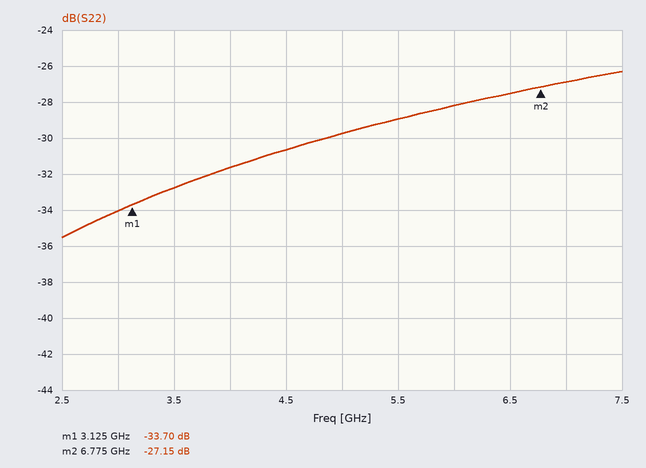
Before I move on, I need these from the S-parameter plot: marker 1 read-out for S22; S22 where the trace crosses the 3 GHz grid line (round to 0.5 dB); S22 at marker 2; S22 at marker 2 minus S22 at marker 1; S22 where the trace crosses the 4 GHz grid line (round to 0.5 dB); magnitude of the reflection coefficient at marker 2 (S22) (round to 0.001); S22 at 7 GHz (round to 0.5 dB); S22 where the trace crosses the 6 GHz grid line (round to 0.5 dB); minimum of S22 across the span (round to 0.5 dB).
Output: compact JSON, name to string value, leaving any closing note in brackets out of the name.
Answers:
{"marker 1 read-out for S22": "-33.70 dB", "S22 where the trace crosses the 3 GHz grid line": "-34.0 dB", "S22 at marker 2": "-27.15 dB", "S22 at marker 2 minus S22 at marker 1": "6.55 dB", "S22 where the trace crosses the 4 GHz grid line": "-31.5 dB", "magnitude of the reflection coefficient at marker 2 (S22)": "0.044", "S22 at 7 GHz": "-27.0 dB", "S22 where the trace crosses the 6 GHz grid line": "-28.0 dB", "minimum of S22 across the span": "-35.5 dB"}
